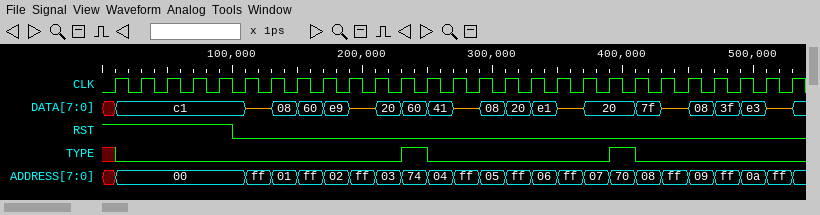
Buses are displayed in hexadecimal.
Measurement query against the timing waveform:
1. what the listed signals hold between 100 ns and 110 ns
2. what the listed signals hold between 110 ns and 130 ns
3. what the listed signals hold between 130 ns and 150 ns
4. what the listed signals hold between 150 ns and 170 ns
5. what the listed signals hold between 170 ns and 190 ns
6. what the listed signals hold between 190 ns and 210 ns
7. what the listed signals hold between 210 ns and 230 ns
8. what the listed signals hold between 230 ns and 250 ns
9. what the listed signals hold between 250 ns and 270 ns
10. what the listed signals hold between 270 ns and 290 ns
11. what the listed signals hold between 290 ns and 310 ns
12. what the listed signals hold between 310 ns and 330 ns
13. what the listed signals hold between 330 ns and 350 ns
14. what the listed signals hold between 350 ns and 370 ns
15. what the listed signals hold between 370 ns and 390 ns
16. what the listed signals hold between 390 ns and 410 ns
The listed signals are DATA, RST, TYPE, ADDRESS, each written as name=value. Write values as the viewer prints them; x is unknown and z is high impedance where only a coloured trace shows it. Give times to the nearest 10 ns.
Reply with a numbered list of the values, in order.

1. DATA=c1, RST=0, TYPE=0, ADDRESS=00
2. DATA=z, RST=0, TYPE=0, ADDRESS=ff
3. DATA=08, RST=0, TYPE=0, ADDRESS=01
4. DATA=60, RST=0, TYPE=0, ADDRESS=ff
5. DATA=e9, RST=0, TYPE=0, ADDRESS=02
6. DATA=z, RST=0, TYPE=0, ADDRESS=ff
7. DATA=20, RST=0, TYPE=0, ADDRESS=03
8. DATA=60, RST=0, TYPE=1, ADDRESS=74
9. DATA=41, RST=0, TYPE=0, ADDRESS=04
10. DATA=z, RST=0, TYPE=0, ADDRESS=ff
11. DATA=08, RST=0, TYPE=0, ADDRESS=05
12. DATA=20, RST=0, TYPE=0, ADDRESS=ff
13. DATA=e1, RST=0, TYPE=0, ADDRESS=06
14. DATA=z, RST=0, TYPE=0, ADDRESS=ff
15. DATA=20, RST=0, TYPE=0, ADDRESS=07
16. DATA=20, RST=0, TYPE=1, ADDRESS=70
